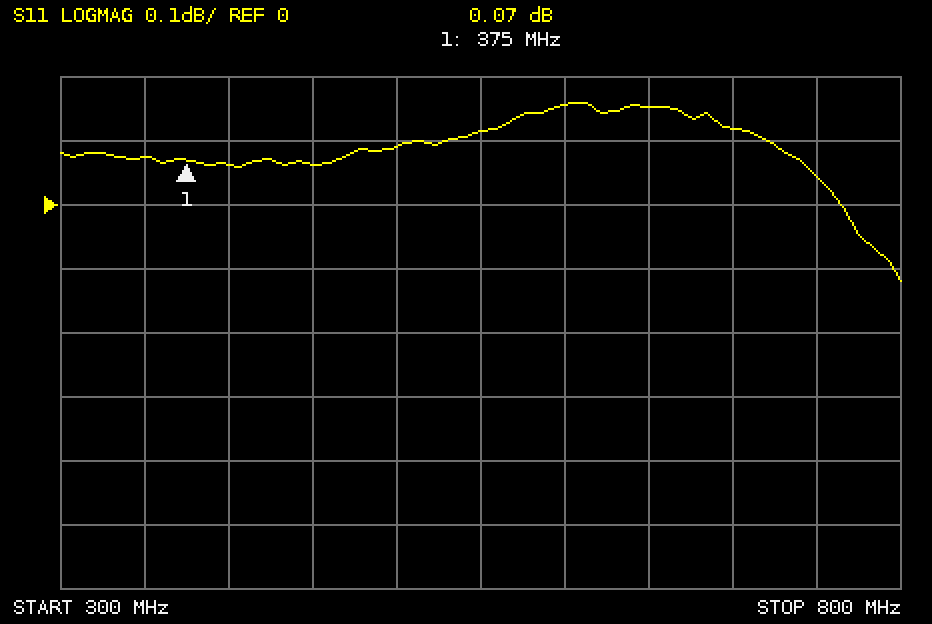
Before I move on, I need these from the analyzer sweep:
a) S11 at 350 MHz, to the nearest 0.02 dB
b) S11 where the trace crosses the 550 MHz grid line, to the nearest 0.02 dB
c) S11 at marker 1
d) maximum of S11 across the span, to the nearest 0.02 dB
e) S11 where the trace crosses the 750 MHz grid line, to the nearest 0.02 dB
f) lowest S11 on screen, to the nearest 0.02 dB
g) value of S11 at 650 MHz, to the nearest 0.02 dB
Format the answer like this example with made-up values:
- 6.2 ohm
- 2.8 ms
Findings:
- 0.08 dB
- 0.12 dB
- 0.07 dB
- 0.16 dB
- 0.04 dB
- -0.12 dB
- 0.16 dB
